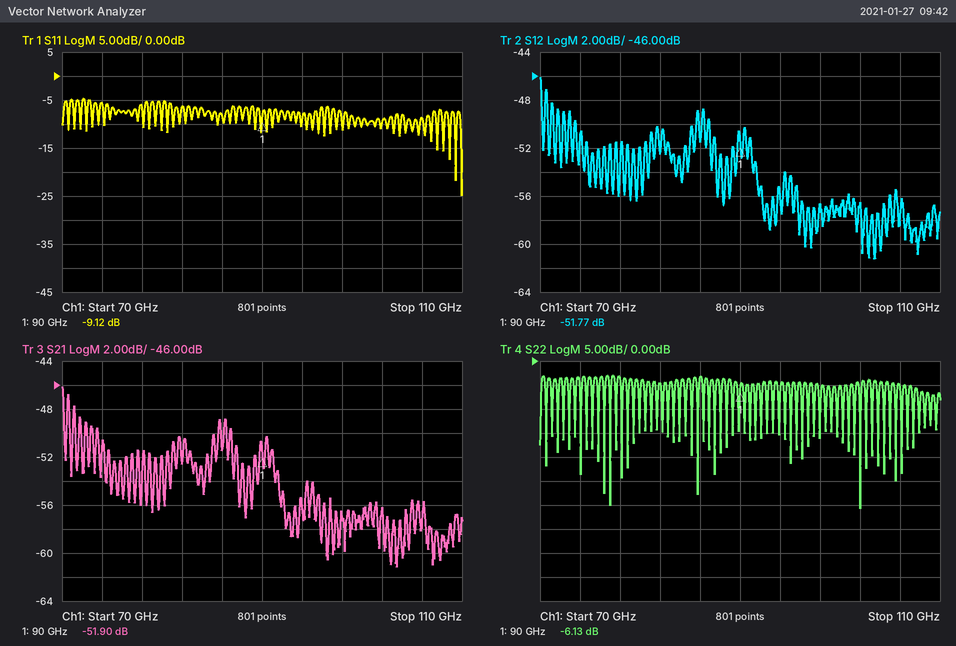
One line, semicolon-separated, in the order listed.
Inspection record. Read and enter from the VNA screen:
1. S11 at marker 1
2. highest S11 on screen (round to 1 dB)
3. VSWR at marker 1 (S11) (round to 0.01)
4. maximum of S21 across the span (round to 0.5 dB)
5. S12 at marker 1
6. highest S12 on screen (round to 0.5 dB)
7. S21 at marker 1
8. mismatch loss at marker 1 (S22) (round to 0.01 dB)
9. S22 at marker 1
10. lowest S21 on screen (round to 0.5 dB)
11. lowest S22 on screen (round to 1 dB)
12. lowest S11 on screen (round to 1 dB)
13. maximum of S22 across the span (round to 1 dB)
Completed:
-9.12 dB; -5 dB; 2.08; -46.0 dB; -51.77 dB; -46.0 dB; -51.90 dB; 1.21 dB; -6.13 dB; -61.0 dB; -31 dB; -25 dB; -3 dB
